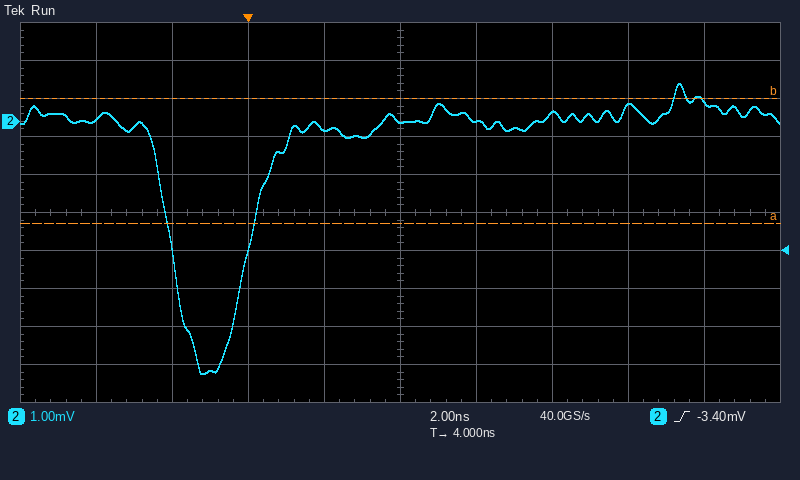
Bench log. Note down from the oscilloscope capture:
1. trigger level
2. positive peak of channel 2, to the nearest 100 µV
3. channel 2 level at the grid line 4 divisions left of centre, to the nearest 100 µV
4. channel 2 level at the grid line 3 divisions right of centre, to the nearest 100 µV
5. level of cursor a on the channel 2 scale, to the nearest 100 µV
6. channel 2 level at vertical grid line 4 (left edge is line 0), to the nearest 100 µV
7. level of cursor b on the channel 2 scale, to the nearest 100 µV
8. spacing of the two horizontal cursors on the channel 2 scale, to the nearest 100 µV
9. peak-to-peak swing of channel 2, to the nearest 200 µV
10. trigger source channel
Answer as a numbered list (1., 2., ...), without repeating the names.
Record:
1. -3.40 mV
2. 1.0 mV
3. 100 µV
4. 400 µV
5. -2.7 mV
6. -200 µV
7. 600 µV
8. 3.3 mV
9. 7.6 mV
10. channel 2
